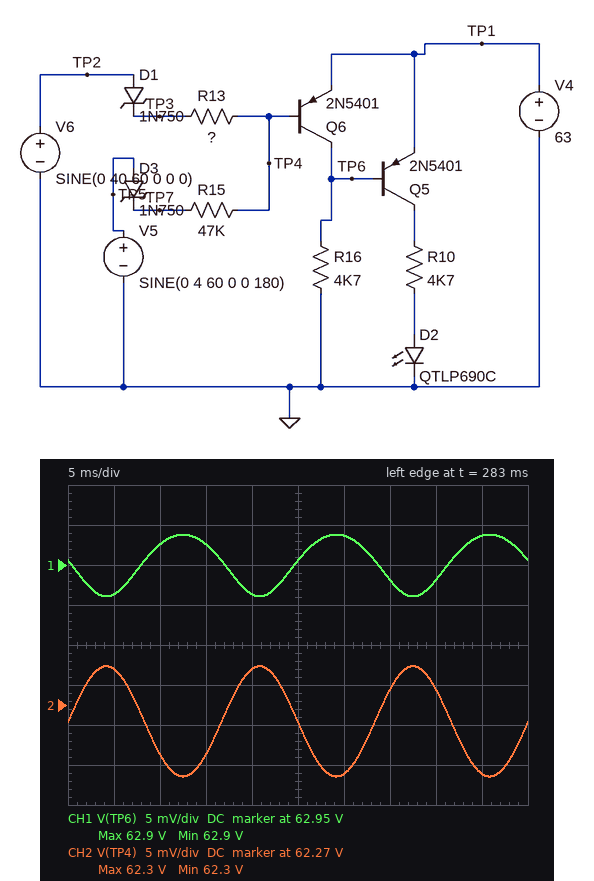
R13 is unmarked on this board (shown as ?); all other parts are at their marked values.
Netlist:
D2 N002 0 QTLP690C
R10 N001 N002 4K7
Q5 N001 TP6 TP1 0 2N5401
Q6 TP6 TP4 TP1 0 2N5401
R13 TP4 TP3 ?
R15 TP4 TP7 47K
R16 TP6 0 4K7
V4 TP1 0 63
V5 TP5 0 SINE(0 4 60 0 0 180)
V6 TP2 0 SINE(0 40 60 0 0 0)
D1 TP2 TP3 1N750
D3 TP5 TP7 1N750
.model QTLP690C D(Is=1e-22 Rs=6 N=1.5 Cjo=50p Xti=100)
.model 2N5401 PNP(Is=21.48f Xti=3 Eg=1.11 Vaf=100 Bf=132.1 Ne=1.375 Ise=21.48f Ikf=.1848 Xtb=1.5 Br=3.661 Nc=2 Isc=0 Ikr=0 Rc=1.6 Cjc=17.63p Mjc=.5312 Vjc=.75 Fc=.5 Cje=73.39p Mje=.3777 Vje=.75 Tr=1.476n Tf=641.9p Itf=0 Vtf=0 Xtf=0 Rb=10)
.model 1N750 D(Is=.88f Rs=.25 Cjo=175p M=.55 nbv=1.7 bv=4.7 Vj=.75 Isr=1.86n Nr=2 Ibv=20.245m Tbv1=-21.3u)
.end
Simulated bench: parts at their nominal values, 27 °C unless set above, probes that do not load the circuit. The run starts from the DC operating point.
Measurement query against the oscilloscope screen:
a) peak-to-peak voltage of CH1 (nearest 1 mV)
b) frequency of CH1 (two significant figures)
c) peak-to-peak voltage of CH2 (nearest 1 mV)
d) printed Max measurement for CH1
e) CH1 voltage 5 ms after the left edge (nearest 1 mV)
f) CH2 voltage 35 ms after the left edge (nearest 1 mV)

8 mV
60 Hz
14 mV
62.9 V
62.941 V
62.267 V
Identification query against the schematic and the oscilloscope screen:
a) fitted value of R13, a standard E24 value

75 kΩ
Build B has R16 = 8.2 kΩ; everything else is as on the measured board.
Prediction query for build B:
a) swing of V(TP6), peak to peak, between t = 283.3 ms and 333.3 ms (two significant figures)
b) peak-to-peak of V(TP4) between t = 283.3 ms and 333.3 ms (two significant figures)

5.7 mV
15 mV
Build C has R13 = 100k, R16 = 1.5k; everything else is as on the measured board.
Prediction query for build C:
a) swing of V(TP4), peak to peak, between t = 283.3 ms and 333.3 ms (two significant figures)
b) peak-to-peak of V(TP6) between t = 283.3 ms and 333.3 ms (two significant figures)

7.8 mV
10 mV
